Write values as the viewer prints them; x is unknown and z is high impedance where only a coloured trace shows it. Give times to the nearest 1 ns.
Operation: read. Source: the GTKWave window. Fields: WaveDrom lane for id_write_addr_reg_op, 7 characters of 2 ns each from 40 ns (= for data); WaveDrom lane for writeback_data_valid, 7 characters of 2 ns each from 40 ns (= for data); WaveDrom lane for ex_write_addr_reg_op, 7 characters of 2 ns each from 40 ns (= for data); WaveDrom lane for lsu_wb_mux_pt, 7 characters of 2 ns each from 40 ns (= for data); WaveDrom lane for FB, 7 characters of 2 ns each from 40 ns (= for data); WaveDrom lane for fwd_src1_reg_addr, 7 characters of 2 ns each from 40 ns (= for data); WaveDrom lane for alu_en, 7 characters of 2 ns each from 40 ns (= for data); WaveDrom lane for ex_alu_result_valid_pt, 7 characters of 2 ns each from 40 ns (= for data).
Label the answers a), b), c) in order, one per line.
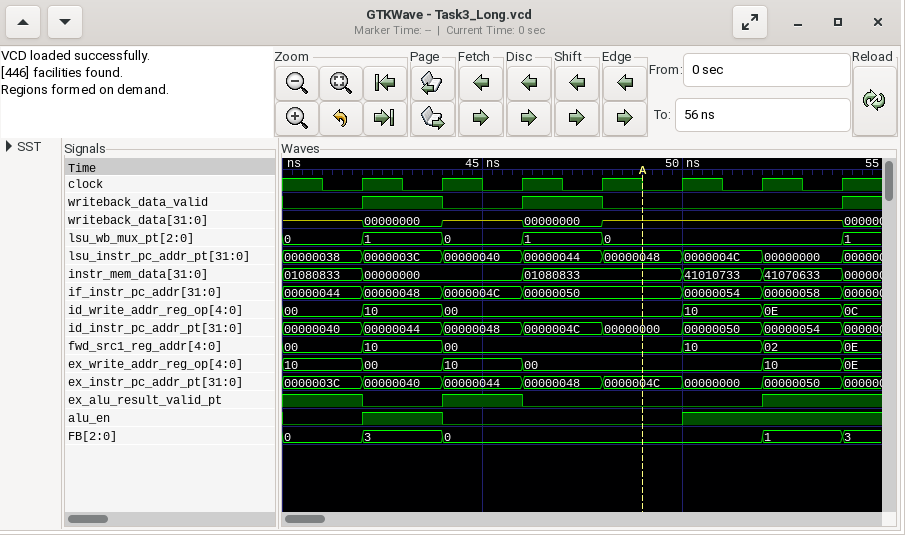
a) {name: 'id_write_addr_reg_op', wave: '===..==', data: '00 10 00 10 0E'}
b) {name: 'writeback_data_valid', wave: '01010..'}
c) {name: 'ex_write_addr_reg_op', wave: '====..=', data: '10 00 10 00 10'}
d) {name: 'lsu_wb_mux_pt', wave: '=====..', data: '0 1 0 1 0'}
e) {name: 'FB', wave: '===...=', data: '0 3 0 1'}
f) {name: 'fwd_src1_reg_addr', wave: '===..==', data: '00 10 00 10 02'}
g) {name: 'alu_en', wave: '010..1.'}
h) {name: 'ex_alu_result_valid_pt', wave: '1010..1'}
